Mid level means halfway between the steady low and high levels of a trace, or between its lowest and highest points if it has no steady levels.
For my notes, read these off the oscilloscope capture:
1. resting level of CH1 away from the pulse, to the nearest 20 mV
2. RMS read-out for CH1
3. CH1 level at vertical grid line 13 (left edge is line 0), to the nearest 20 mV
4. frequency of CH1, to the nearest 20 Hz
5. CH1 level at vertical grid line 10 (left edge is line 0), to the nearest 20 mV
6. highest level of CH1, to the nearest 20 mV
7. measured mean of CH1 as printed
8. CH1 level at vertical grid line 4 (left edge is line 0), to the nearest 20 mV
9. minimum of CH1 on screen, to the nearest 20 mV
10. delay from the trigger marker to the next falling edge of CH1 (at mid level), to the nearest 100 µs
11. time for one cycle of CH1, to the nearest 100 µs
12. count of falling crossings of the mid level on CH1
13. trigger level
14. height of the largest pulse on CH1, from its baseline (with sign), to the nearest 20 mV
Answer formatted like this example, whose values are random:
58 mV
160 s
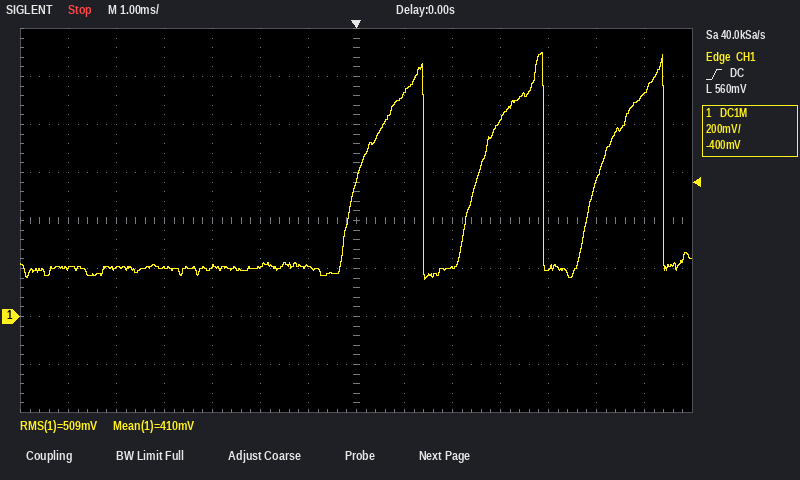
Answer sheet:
200 mV
509 mV
920 mV
400 Hz
820 mV
1.10 V
410 mV
200 mV
160 mV
1.4 ms
2.5 ms
3
560 mV
+900 mV
